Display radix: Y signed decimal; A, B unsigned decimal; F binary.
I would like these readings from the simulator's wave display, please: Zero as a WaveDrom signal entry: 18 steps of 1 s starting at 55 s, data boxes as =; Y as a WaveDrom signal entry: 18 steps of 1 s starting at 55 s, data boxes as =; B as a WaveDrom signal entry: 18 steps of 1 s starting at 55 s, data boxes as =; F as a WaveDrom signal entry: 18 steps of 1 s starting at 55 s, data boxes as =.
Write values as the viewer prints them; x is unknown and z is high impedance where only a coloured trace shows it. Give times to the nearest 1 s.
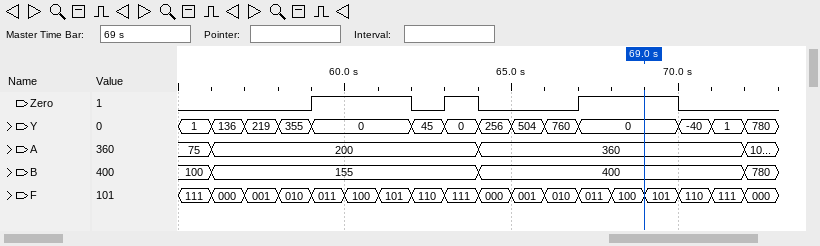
{name: 'Zero', wave: '0...1..010..1..0..'}
{name: 'Y', wave: '=====..======..===', data: '1 136 219 355 0 45 0 256 504 760 0 -40 1 780'}
{name: 'B', wave: '==.......=.......=', data: '100 155 400 780'}
{name: 'F', wave: '==================', data: '111 000 001 010 011 100 101 110 111 000 001 010 011 100 101 110 111 000'}
